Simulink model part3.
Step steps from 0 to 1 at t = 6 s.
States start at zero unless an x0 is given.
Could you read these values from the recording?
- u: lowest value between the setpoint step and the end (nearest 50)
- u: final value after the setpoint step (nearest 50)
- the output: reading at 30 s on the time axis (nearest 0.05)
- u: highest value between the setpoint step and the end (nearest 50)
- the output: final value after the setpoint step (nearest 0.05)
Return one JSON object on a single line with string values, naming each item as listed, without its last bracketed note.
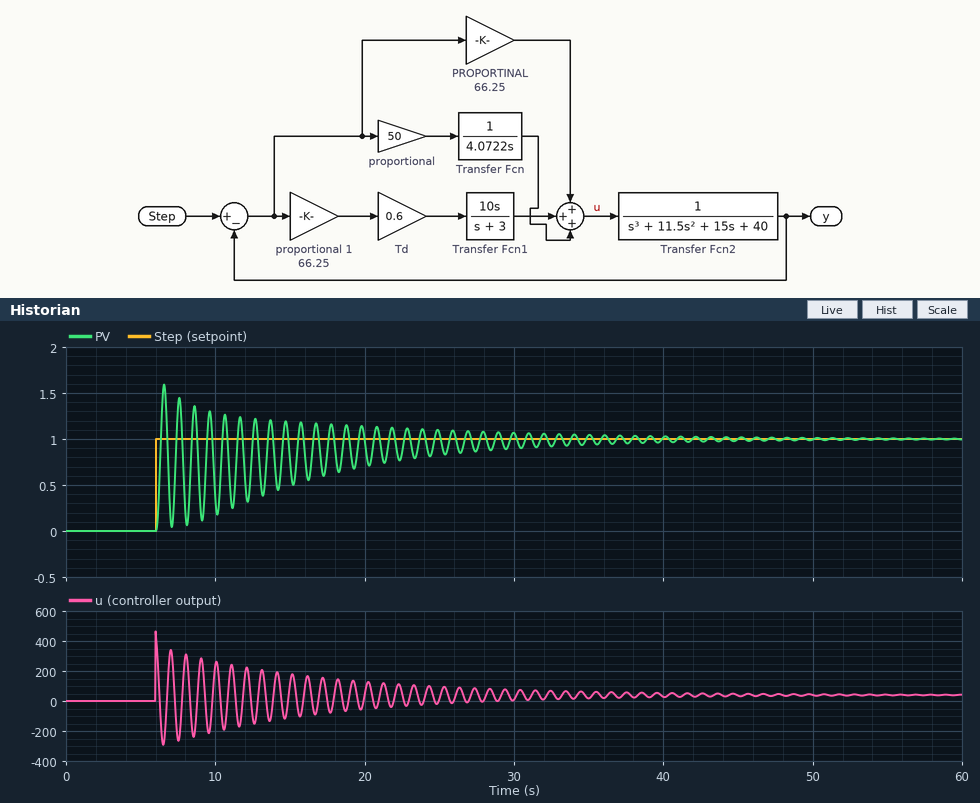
{"u: lowest value between the setpoint step and the end": "-300", "u: final value after the setpoint step": "50", "the output: reading at 30 s on the time axis": "1.05", "u: highest value between the setpoint step and the end": "450", "the output: final value after the setpoint step": "1.00"}
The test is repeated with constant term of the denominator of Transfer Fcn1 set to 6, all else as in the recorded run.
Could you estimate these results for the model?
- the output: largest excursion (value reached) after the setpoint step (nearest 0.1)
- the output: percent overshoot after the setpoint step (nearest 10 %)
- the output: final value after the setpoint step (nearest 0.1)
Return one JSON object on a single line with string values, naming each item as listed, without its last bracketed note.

{"the output: largest excursion (value reached) after the setpoint step": "1.3", "the output: percent overshoot after the setpoint step": "30 %", "the output: final value after the setpoint step": "1.0"}
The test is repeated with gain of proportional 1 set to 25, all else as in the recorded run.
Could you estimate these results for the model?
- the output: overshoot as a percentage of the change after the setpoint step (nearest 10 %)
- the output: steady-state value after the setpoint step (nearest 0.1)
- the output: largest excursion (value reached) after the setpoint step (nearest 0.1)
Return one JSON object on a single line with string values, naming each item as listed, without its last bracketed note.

{"the output: overshoot as a percentage of the change after the setpoint step": "30 %", "the output: steady-state value after the setpoint step": "1.0", "the output: largest excursion (value reached) after the setpoint step": "1.3"}
